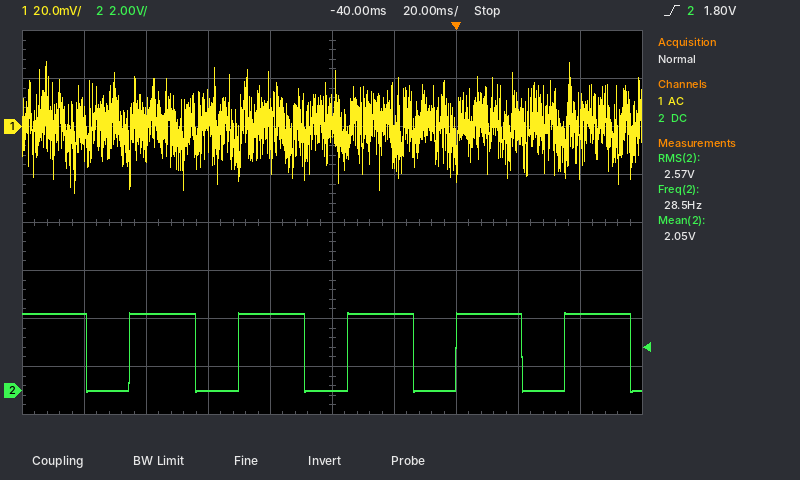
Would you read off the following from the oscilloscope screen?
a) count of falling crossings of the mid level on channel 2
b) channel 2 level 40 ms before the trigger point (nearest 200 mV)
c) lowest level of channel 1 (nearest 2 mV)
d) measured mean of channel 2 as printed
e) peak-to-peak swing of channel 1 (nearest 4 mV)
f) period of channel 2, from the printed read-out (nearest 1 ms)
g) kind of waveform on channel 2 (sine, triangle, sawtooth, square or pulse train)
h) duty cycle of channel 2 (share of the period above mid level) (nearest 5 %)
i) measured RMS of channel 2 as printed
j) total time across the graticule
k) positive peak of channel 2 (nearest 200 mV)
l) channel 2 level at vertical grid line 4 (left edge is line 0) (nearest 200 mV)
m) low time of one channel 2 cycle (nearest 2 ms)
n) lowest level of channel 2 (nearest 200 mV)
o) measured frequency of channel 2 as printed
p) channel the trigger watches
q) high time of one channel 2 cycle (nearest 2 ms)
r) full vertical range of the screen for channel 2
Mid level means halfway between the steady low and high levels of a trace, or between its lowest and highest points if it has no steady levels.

6
0.0 V
-28 mV
2.05 V
56 mV
35 ms
pulse train
60 %
2.57 V
200 ms
3.2 V
3.2 V
14 ms
0.0 V
28.5 Hz
channel 2
22 ms
16 V
